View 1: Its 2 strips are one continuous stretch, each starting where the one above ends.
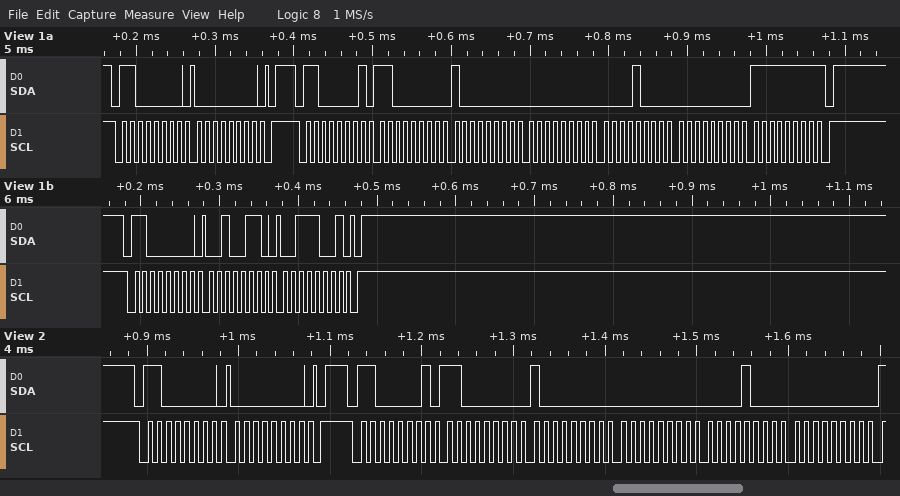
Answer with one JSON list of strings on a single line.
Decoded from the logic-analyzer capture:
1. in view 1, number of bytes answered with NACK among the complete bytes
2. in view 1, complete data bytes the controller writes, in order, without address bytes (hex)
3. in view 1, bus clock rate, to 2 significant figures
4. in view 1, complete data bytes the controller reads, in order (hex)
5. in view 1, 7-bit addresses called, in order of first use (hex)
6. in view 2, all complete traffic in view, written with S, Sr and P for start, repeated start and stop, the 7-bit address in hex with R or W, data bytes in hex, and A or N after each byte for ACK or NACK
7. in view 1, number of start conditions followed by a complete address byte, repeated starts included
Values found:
["1", "00 26 39", "100 kHz", "C0 80 00 08 00 FF", "0x60", "S 60W A 00 A P S 60R A C0 A 80 A 00 A 08 A 00 A", "3"]
